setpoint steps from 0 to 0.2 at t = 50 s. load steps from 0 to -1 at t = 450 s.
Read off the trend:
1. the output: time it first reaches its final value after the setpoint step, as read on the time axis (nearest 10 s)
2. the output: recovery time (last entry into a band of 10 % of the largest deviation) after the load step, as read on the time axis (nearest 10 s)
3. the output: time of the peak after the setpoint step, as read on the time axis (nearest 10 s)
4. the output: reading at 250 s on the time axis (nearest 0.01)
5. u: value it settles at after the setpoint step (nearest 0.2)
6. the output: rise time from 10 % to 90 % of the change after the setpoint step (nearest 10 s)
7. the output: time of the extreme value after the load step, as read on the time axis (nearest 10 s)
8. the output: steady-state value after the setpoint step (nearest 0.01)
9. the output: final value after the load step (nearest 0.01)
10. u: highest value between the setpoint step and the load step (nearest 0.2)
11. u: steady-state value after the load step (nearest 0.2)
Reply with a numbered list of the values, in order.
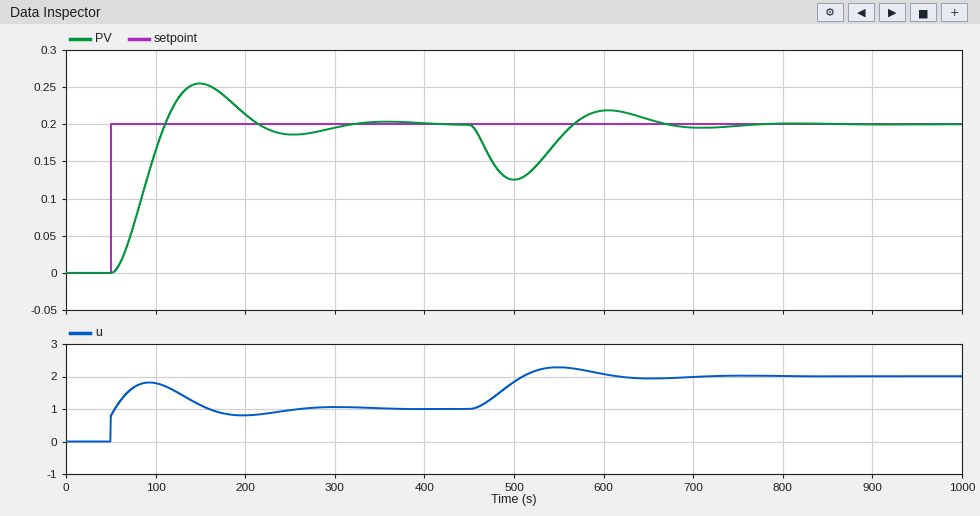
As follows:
1. 110 s
2. 650 s
3. 150 s
4. 0.19
5. 1.0
6. 40 s
7. 500 s
8. 0.20
9. 0.20
10. 1.8
11. 2.0
